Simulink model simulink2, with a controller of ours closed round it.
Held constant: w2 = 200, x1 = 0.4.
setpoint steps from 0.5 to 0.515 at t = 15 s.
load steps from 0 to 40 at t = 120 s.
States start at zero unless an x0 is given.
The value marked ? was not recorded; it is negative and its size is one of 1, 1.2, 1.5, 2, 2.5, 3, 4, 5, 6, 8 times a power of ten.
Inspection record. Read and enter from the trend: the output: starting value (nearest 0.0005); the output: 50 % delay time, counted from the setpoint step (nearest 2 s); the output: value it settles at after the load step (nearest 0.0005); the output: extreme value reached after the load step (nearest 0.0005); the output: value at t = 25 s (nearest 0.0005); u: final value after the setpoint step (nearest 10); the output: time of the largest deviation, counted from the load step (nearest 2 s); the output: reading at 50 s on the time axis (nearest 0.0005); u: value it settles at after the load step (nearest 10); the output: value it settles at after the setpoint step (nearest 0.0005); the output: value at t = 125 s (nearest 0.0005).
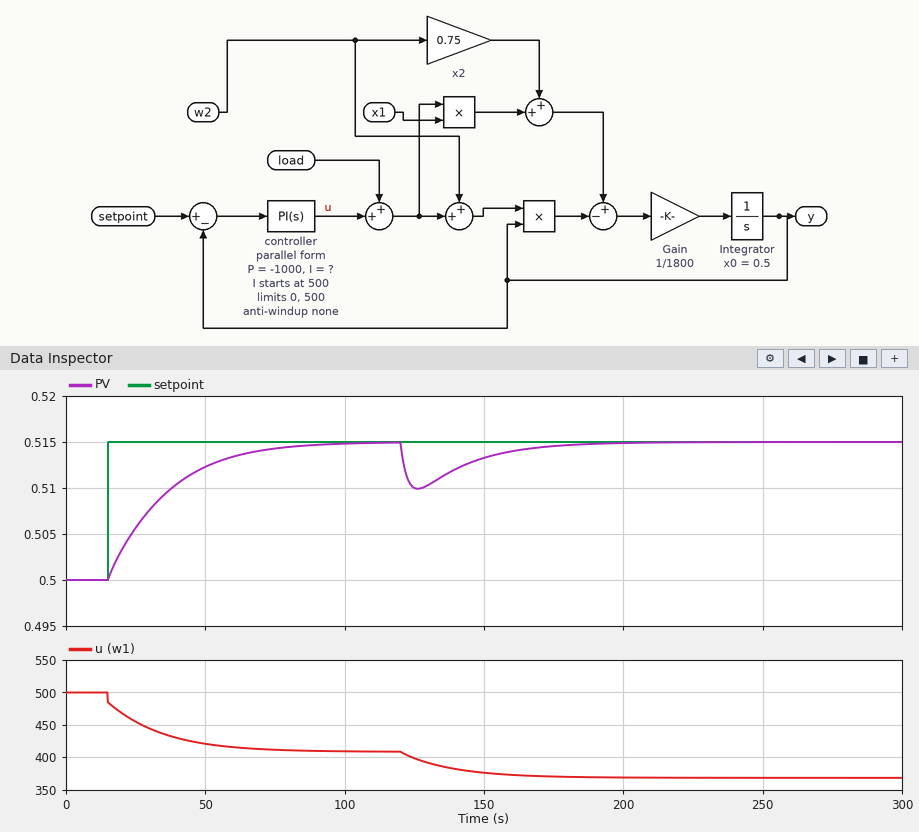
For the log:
0.5000
14 s
0.5150
0.5100
0.5055
410
6 s
0.5125
370
0.5150
0.5100
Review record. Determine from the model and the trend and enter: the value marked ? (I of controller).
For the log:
-300
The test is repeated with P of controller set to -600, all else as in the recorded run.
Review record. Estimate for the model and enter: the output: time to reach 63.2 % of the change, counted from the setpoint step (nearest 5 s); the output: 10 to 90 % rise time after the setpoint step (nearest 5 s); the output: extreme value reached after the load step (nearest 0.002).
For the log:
20 s
40 s
0.510
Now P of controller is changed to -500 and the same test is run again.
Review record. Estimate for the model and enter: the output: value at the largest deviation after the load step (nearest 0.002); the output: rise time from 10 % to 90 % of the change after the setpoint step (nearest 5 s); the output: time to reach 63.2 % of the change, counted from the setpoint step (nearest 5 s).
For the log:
0.510
40 s
20 s
